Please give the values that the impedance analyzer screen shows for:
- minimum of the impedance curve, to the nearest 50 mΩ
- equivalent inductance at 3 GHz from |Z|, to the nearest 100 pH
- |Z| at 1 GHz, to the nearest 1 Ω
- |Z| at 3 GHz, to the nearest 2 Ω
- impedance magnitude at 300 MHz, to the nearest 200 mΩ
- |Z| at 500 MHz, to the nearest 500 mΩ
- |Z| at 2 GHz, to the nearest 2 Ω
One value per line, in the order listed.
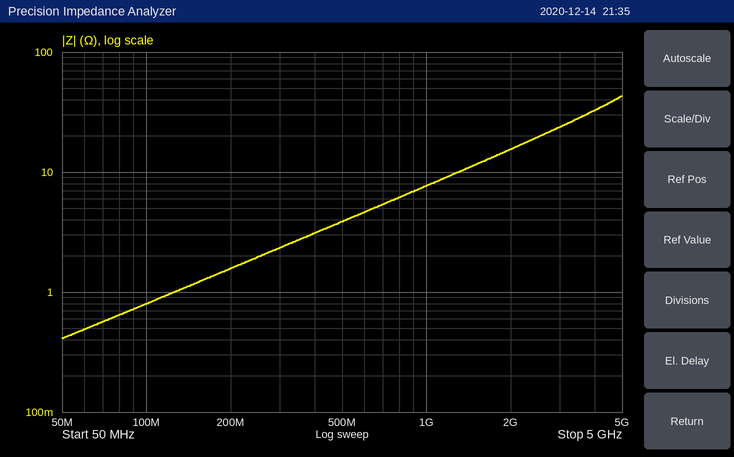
400 mΩ
1.3 nH
8 Ω
24 Ω
2.4 Ω
4.0 Ω
16 Ω
